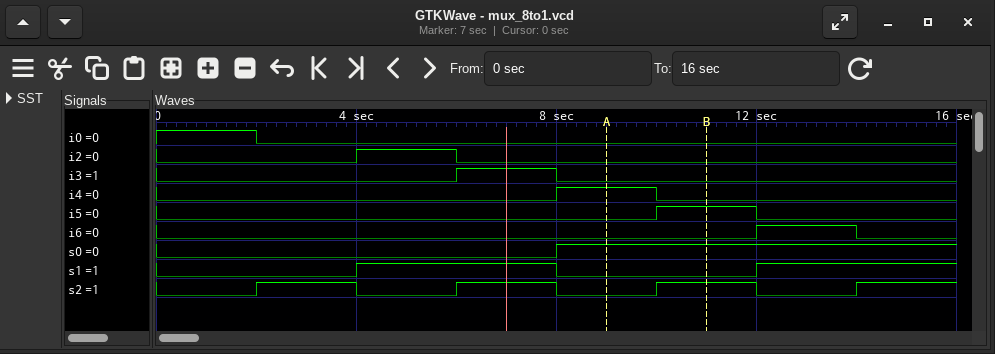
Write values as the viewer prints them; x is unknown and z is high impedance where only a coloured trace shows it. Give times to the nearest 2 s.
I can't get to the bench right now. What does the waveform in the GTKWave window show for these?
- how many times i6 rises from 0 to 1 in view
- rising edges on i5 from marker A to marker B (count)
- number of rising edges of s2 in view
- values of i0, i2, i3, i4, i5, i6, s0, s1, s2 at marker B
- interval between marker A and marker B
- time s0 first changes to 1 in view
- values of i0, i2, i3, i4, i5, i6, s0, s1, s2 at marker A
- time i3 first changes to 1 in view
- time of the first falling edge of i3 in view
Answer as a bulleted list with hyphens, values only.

- 1
- 1
- 4
- i0=0, i2=0, i3=0, i4=0, i5=1, i6=0, s0=1, s1=0, s2=1
- 2 s
- 8 s
- i0=0, i2=0, i3=0, i4=1, i5=0, i6=0, s0=1, s1=0, s2=0
- 6 s
- 8 s
